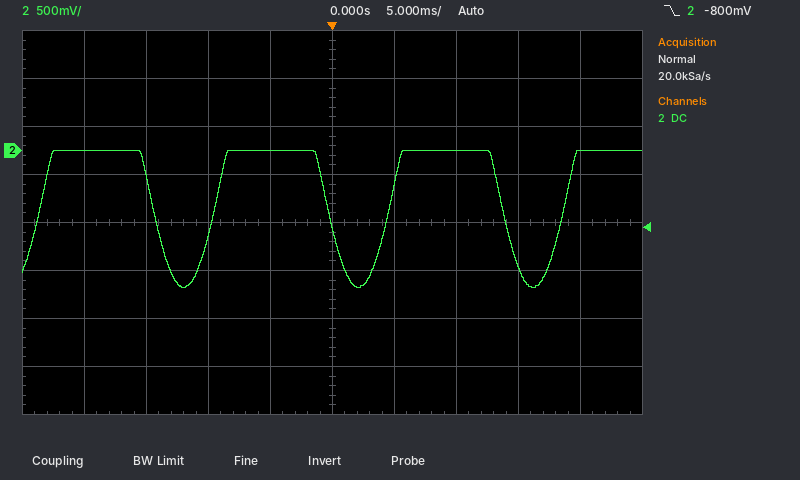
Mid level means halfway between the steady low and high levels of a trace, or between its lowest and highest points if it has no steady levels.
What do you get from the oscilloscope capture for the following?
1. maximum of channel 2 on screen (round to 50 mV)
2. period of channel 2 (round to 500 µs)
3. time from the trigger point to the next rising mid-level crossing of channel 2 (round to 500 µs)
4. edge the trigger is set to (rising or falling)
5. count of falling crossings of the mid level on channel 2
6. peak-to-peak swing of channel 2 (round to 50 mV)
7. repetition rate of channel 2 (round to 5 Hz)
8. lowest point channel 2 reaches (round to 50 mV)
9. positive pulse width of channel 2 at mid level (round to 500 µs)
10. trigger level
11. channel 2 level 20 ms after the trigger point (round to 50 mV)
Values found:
0 mV
14.0 ms
4.5 ms
falling
3
1.45 V
70 Hz
-1.45 V
9.5 ms
-800 mV
0 mV
